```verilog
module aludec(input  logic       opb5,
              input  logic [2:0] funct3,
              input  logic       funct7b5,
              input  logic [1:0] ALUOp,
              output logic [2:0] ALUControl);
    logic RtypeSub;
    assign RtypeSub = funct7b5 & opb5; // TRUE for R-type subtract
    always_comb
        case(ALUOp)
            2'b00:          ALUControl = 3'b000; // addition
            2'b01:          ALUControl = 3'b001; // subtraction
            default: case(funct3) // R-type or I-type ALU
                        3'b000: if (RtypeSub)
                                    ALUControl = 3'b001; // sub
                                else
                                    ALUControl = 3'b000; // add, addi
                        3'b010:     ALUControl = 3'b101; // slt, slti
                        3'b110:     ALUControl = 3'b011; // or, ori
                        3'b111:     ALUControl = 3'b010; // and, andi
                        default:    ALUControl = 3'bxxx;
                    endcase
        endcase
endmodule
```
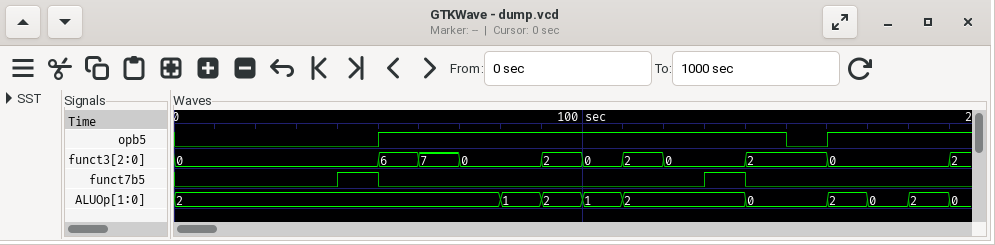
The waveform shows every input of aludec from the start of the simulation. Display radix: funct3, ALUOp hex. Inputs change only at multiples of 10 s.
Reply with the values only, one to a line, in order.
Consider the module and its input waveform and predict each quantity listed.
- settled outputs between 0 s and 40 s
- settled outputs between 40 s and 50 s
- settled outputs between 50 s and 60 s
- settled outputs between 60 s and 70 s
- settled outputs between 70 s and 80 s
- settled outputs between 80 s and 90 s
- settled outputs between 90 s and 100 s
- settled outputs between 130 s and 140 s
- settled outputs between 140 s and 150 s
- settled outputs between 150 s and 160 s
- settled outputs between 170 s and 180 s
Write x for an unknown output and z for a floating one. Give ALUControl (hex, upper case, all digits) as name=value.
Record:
ALUControl=0
ALUControl=0
ALUControl=3
ALUControl=2
ALUControl=0
ALUControl=1
ALUControl=5
ALUControl=1
ALUControl=0
ALUControl=0
ALUControl=0
